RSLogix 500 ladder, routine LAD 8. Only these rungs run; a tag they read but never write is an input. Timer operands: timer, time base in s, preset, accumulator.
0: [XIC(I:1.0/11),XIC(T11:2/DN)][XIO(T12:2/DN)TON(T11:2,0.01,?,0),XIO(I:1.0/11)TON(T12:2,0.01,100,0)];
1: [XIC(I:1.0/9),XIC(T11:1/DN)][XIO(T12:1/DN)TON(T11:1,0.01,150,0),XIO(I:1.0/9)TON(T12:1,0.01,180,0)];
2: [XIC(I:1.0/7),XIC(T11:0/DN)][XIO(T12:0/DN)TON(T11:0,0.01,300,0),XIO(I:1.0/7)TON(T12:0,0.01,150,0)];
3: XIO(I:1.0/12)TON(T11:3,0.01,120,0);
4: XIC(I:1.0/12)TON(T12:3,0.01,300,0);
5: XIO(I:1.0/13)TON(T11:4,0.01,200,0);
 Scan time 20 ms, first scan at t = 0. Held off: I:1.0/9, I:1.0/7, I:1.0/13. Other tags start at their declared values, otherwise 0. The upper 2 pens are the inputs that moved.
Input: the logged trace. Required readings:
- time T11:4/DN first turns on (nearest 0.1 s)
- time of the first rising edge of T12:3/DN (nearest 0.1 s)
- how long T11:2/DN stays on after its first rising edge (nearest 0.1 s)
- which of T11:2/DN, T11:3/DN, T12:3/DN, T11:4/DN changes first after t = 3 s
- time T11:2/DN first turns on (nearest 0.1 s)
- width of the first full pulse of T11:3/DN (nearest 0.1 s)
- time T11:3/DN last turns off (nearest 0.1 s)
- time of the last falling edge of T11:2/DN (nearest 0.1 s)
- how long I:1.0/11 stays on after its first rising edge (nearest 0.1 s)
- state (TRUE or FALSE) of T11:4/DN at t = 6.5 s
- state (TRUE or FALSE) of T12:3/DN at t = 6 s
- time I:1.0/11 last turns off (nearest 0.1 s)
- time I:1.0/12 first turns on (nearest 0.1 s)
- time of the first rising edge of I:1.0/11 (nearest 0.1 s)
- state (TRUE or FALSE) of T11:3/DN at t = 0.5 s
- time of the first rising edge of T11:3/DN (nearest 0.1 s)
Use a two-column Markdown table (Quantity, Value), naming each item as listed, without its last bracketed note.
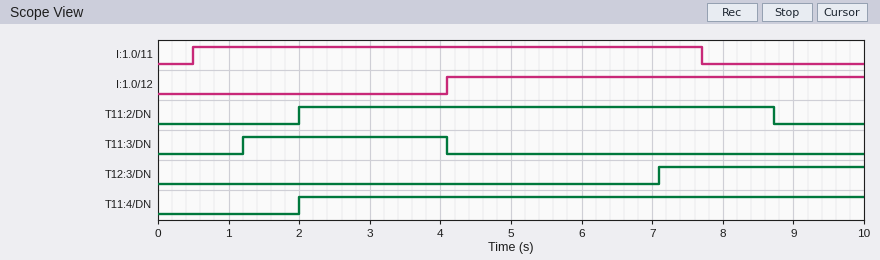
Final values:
| Quantity | Value |
|---|---|
| time T11:4/DN first turns on | 2.0 s |
| time of the first rising edge of T12:3/DN | 7.1 s |
| how long T11:2/DN stays on after its first rising edge | 6.7 s |
| which of T11:2/DN, T11:3/DN, T12:3/DN, T11:4/DN changes first after t = 3 s | T11:3/DN |
| time T11:2/DN first turns on | 2.0 s |
| width of the first full pulse of T11:3/DN | 2.9 s |
| time T11:3/DN last turns off | 4.1 s |
| time of the last falling edge of T11:2/DN | 8.7 s |
| how long I:1.0/11 stays on after its first rising edge | 7.2 s |
| state (TRUE or FALSE) of T11:4/DN at t = 6.5 s | TRUE |
| state (TRUE or FALSE) of T12:3/DN at t = 6 s | FALSE |
| time I:1.0/11 last turns off | 7.7 s |
| time I:1.0/12 first turns on | 4.1 s |
| time of the first rising edge of I:1.0/11 | 0.5 s |
| state (TRUE or FALSE) of T11:3/DN at t = 0.5 s | FALSE |
| time of the first rising edge of T11:3/DN | 1.2 s |
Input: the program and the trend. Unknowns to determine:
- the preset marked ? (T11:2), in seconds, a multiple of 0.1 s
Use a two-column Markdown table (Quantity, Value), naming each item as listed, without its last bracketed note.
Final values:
| Quantity | Value |
|---|---|
| the preset marked ? (T11:2), in seconds, a multiple of 0.1 s | 1.5 s |
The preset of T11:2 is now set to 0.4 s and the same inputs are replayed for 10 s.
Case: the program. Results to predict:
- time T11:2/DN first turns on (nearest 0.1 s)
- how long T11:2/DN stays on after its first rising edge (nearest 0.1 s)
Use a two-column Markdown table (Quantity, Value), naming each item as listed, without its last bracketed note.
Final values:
| Quantity | Value |
|---|---|
| time T11:2/DN first turns on | 0.9 s |
| how long T11:2/DN stays on after its first rising edge | 7.8 s |
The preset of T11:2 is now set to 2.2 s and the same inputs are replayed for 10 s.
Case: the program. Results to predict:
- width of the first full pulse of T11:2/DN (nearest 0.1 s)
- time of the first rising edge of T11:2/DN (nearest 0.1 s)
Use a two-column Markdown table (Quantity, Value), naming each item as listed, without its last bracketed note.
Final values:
| Quantity | Value |
|---|---|
| width of the first full pulse of T11:2/DN | 6.0 s |
| time of the first rising edge of T11:2/DN | 2.7 s |
